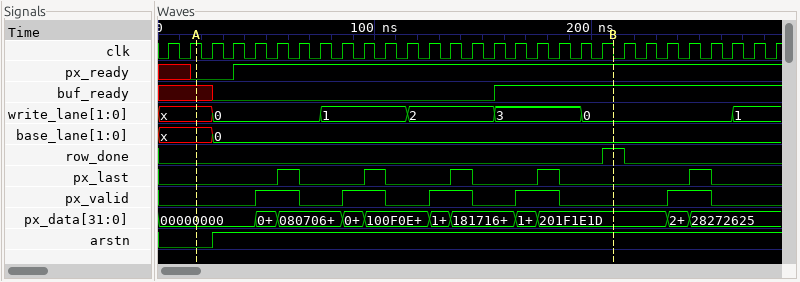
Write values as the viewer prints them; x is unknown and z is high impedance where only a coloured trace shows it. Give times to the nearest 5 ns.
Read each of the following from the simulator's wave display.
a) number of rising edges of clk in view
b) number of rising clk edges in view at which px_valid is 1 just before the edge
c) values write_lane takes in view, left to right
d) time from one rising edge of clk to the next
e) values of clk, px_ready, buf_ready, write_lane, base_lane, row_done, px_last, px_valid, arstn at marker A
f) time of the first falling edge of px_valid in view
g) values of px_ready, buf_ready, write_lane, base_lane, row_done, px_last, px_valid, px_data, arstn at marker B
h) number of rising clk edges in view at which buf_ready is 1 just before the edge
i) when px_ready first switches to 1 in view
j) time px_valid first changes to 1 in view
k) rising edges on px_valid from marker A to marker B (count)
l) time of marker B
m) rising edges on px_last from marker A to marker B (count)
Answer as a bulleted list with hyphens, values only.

- 29
- 10
- x, 0, 1, 2, 3, 0, 1
- 10 ns
- clk=1, px_ready=0, buf_ready=x, write_lane=x, base_lane=x, row_done=0, px_last=0, px_valid=0, arstn=0
- 65 ns
- px_ready=1, buf_ready=1, write_lane=0, base_lane=0, row_done=1, px_last=0, px_valid=0, px_data=201F1E1D, arstn=1
- 13
- 35 ns
- 45 ns
- 4
- 210 ns
- 4
